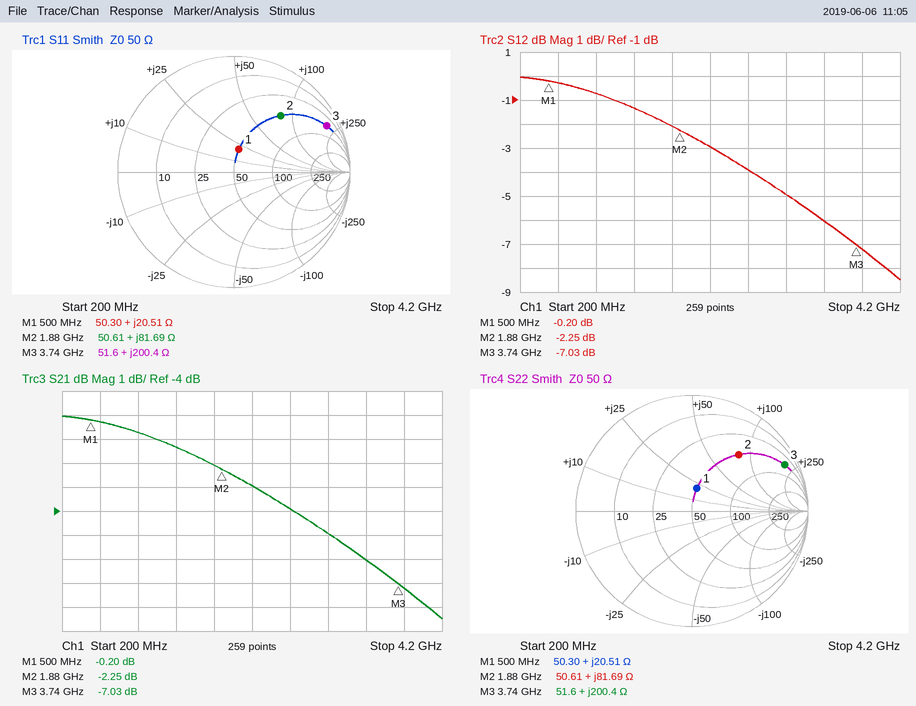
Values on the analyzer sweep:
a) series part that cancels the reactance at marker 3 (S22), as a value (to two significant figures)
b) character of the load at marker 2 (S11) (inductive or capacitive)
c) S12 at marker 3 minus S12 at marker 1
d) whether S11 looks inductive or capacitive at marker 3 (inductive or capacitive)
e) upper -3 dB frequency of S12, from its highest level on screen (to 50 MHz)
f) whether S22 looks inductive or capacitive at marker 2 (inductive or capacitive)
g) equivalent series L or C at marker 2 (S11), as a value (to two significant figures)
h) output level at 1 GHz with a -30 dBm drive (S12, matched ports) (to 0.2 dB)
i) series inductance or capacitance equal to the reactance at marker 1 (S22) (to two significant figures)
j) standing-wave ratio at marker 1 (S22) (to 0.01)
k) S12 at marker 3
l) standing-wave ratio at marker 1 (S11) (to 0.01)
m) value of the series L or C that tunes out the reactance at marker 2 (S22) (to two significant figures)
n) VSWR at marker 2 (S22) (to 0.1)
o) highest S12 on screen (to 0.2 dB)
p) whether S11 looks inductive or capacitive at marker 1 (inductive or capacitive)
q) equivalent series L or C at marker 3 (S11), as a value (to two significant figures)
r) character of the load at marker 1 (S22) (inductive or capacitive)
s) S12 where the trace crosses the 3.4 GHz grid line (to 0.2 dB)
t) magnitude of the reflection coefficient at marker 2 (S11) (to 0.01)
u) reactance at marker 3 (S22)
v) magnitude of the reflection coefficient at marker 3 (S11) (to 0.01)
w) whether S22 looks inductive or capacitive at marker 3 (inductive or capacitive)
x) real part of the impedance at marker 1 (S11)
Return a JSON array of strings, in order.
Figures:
["210 fF", "inductive", "-6.83 dB", "inductive", "2.25 GHz", "inductive", "6.9 nH", "-30.8 dBm", "6.5 nH", "1.50", "-7.03 dB", "1.50", "1.0 pF", "4.4", "0.0 dB", "inductive", "8.5 nH", "inductive", "-6.0 dB", "0.63", "+200.4 Ω", "0.89", "inductive", "50.30 Ω"]
